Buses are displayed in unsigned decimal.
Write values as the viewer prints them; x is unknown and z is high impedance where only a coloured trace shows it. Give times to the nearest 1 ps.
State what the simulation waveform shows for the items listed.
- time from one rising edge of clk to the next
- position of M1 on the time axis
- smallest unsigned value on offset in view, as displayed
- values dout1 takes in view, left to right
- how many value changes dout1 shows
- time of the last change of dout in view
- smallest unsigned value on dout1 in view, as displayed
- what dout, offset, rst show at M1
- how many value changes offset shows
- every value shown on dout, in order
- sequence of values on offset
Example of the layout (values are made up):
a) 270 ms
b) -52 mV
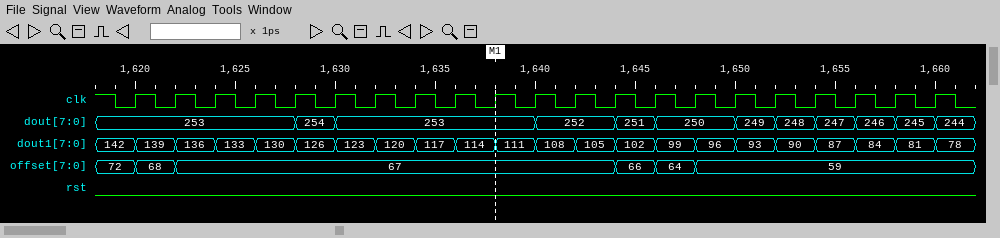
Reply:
a) 2 ps
b) 1638 ps
c) 59
d) 142, 139, 136, 133, 130, 126, 123, 120, 117, 114, 111, 108, 105, 102, 99, 96, 93, 90, 87, 84, 81, 78
e) 21
f) 1660 ps
g) 78
h) dout=253, offset=67, rst=0
i) 5
j) 253, 254, 253, 252, 251, 250, 249, 248, 247, 246, 245, 244
k) 72, 68, 67, 66, 64, 59
